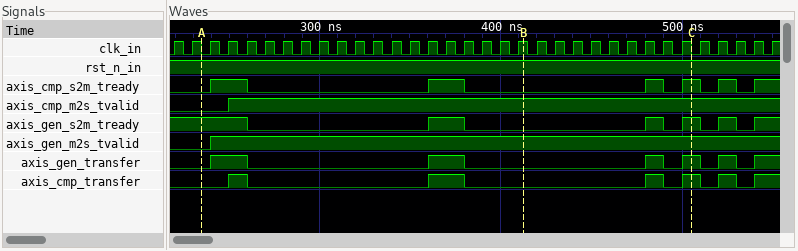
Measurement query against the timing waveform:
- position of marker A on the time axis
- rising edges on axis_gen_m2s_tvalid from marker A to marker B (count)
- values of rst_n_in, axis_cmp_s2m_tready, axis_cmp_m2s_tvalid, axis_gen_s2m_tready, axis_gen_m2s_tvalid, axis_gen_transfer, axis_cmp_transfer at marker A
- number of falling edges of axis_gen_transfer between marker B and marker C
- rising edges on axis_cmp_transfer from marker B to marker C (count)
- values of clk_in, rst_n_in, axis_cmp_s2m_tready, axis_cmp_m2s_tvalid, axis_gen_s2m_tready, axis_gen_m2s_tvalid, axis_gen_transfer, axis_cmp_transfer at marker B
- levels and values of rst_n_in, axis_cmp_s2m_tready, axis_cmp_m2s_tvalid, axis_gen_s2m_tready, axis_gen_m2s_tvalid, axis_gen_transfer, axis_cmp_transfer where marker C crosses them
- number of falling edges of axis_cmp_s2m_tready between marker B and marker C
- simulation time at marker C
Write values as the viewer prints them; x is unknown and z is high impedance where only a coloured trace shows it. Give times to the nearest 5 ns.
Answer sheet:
235 ns
1
rst_n_in=1, axis_cmp_s2m_tready=0, axis_cmp_m2s_tvalid=0, axis_gen_s2m_tready=1, axis_gen_m2s_tvalid=0, axis_gen_transfer=0, axis_cmp_transfer=0
1
2
clk_in=1, rst_n_in=1, axis_cmp_s2m_tready=0, axis_cmp_m2s_tvalid=1, axis_gen_s2m_tready=0, axis_gen_m2s_tvalid=1, axis_gen_transfer=0, axis_cmp_transfer=0
rst_n_in=1, axis_cmp_s2m_tready=1, axis_cmp_m2s_tvalid=1, axis_gen_s2m_tready=1, axis_gen_m2s_tvalid=1, axis_gen_transfer=1, axis_cmp_transfer=1
1
505 ns
